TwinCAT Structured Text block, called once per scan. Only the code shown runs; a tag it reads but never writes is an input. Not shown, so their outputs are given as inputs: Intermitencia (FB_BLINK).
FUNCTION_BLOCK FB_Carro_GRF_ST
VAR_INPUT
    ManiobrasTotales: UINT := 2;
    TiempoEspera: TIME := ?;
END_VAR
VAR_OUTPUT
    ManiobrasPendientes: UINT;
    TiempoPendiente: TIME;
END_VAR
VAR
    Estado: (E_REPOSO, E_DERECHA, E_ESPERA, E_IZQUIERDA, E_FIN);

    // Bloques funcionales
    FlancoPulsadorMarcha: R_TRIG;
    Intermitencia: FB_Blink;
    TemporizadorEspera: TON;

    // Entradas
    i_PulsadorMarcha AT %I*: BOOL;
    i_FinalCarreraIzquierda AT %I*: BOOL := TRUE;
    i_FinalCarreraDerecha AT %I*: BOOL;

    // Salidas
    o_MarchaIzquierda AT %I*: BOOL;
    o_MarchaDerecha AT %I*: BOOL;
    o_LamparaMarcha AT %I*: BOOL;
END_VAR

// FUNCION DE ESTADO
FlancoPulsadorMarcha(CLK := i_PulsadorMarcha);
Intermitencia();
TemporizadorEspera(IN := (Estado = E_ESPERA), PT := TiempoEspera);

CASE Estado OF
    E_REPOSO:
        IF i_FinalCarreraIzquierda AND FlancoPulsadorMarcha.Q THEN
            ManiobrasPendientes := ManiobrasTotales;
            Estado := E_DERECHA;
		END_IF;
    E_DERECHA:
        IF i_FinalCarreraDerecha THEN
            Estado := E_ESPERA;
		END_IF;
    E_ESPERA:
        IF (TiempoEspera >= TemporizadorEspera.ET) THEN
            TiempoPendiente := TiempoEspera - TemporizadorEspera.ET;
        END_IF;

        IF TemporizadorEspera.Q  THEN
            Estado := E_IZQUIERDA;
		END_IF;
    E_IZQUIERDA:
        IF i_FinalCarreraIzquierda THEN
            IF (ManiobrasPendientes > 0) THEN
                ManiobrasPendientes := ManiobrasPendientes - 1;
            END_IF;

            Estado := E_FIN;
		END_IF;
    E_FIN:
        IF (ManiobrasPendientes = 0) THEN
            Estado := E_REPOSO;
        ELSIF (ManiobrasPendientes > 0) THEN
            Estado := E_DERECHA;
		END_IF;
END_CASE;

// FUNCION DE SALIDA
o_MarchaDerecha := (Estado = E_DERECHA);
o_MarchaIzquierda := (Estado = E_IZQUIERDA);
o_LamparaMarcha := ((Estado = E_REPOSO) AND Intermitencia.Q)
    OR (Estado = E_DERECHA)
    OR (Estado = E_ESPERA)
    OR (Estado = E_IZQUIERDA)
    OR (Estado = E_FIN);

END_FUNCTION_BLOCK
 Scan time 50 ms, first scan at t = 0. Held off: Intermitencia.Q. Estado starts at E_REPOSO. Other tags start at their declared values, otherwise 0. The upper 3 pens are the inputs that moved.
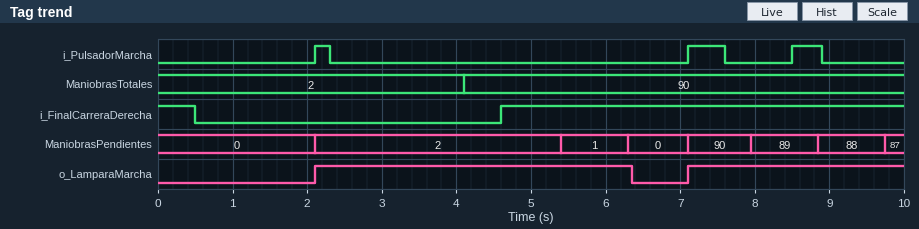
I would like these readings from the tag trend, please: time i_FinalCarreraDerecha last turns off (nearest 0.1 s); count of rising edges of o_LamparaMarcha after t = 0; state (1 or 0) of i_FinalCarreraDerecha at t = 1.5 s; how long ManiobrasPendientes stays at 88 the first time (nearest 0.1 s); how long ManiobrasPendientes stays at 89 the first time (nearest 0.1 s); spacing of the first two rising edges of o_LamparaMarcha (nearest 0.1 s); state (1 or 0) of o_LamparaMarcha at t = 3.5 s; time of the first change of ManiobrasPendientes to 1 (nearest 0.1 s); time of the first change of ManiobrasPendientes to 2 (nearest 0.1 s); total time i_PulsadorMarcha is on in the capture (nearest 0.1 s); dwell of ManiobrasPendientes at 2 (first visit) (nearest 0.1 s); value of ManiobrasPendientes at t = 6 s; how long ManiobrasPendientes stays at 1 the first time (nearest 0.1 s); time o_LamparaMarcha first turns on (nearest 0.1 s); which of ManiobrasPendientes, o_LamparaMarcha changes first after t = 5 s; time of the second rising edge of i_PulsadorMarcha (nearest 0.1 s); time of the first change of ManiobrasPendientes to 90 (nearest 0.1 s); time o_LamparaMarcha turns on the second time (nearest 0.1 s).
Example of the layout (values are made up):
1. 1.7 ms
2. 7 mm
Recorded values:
1. 0.5 s
2. 2
3. 0
4. 0.9 s
5. 0.9 s
6. 5.0 s
7. 1
8. 5.4 s
9. 2.1 s
10. 1.1 s
11. 3.3 s
12. 1
13. 0.9 s
14. 2.1 s
15. ManiobrasPendientes
16. 7.1 s
17. 7.1 s
18. 7.1 s
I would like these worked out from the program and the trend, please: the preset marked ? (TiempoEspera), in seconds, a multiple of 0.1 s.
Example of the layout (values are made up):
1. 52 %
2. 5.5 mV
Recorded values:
1. 0.7 s
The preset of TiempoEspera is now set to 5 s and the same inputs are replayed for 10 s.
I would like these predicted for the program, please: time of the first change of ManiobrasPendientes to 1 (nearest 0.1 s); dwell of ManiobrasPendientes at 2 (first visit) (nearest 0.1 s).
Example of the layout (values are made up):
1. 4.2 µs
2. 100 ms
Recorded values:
1. 9.7 s
2. 7.6 s
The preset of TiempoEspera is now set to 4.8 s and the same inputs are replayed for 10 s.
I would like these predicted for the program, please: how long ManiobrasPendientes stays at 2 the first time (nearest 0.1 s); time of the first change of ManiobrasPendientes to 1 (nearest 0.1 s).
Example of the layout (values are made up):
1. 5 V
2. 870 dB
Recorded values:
1. 7.4 s
2. 9.5 s
